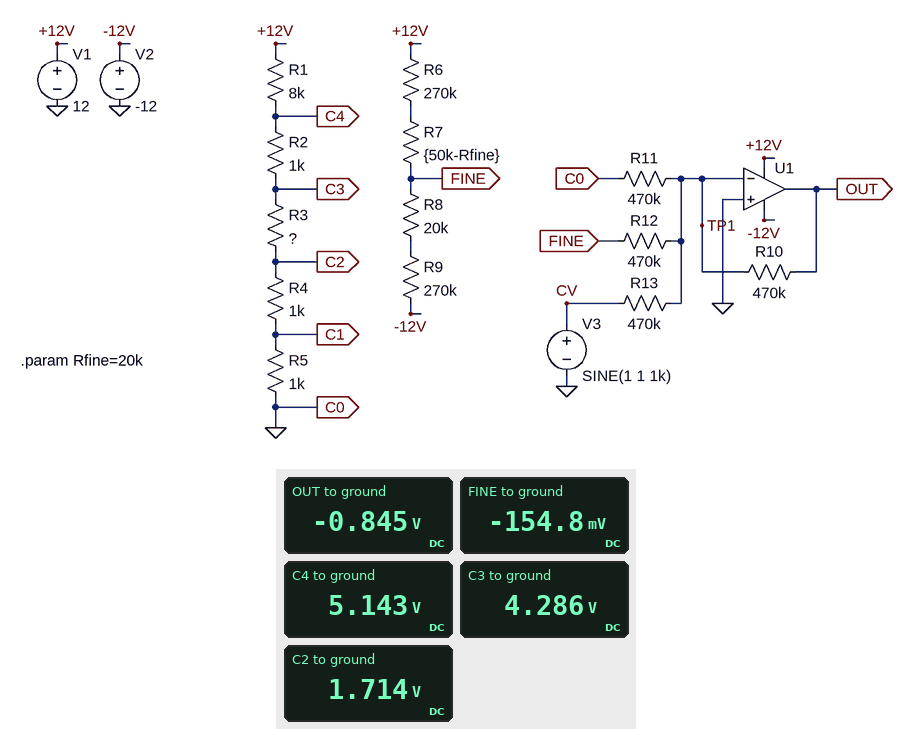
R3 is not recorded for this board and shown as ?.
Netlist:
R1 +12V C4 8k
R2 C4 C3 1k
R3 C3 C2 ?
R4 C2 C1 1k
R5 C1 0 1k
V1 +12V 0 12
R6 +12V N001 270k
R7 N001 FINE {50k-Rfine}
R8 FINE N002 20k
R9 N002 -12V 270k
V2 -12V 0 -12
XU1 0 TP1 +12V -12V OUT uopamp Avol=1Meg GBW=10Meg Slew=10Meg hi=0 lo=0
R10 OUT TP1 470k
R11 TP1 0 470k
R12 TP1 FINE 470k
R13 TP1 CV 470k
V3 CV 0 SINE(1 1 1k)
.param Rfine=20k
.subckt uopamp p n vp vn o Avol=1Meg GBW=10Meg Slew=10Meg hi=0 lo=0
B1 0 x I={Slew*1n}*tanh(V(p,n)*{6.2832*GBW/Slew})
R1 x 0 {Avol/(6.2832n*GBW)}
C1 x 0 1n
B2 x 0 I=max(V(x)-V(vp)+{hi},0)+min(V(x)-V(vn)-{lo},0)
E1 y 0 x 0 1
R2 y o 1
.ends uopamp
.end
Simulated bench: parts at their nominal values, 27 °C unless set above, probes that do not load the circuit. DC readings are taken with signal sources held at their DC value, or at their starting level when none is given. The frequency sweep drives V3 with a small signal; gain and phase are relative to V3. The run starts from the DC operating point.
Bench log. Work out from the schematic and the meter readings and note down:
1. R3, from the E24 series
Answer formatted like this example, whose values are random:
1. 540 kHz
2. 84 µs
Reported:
1. 3 kΩ
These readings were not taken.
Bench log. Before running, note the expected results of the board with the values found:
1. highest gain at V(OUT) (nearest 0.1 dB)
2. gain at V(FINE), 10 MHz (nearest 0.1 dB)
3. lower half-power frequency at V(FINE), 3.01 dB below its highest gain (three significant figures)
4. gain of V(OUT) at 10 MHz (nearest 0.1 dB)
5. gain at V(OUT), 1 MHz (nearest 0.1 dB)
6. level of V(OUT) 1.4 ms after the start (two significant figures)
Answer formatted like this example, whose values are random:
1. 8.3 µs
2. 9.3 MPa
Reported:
1. 0 dB
2. -24.2 dB
3. 2.66 MHz
4. -11.8 dB
5. -0.6 dB
6. -1.4 V
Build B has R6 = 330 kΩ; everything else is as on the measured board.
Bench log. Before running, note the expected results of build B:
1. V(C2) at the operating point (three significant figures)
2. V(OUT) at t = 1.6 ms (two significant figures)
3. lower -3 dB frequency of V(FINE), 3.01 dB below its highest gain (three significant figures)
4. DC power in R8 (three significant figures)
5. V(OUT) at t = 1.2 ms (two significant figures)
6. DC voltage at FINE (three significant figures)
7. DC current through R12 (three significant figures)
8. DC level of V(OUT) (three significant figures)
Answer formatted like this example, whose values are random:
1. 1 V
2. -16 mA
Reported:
1. 1.71 V
2. 550 mV
3. 2.67 MHz
4. 29.0 µW
5. -990 mV
6. -963 mV
7. 2.05 µA
8. -36.8 mV
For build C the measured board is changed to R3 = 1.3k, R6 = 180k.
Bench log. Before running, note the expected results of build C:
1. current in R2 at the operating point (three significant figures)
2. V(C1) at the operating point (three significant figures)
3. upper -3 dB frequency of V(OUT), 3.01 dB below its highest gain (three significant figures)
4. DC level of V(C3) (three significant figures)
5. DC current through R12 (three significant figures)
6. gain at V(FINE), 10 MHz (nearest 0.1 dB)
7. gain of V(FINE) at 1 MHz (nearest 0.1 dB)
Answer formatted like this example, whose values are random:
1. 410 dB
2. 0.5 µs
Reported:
1. 976 µA
2. 976 mV
3. 2.64 MHz
4. 3.22 V
5. 3.24 µA
6. -25.6 dB
7. -34.3 dB
